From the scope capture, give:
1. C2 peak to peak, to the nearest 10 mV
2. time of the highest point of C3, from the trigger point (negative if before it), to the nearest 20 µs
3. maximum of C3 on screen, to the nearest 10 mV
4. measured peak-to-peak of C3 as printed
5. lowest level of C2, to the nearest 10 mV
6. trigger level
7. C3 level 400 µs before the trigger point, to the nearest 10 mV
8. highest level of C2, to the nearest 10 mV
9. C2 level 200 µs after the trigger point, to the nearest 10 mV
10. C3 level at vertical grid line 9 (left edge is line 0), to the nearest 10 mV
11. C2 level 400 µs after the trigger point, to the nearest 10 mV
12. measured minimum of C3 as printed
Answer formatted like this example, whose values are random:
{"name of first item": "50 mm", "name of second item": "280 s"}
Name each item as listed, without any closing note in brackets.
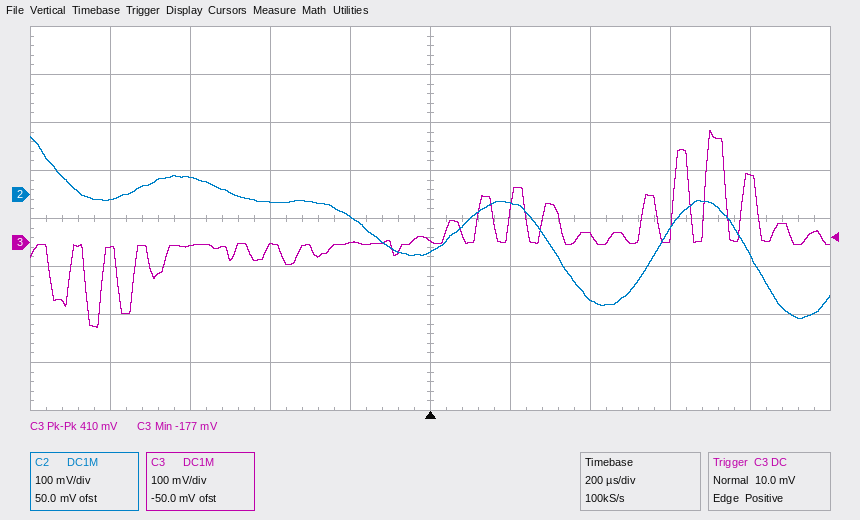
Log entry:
{"C2 peak to peak, to the nearest 10 mV": "380 mV", "time of the highest point of C3, from the trigger point (negative if before it), to the nearest 20 µs": "+700 µs", "maximum of C3 on screen, to the nearest 10 mV": "230 mV", "measured peak-to-peak of C3 as printed": "410 mV", "lowest level of C2, to the nearest 10 mV": "-260 mV", "trigger level": "10.0 mV", "C3 level 400 µs before the trigger point, to the nearest 10 mV": "-10 mV", "highest level of C2, to the nearest 10 mV": "120 mV", "C2 level 200 µs after the trigger point, to the nearest 10 mV": "-20 mV", "C3 level at vertical grid line 9 (left edge is line 0), to the nearest 10 mV": "140 mV", "C2 level 400 µs after the trigger point, to the nearest 10 mV": "-220 mV", "measured minimum of C3 as printed": "-177 mV"}
